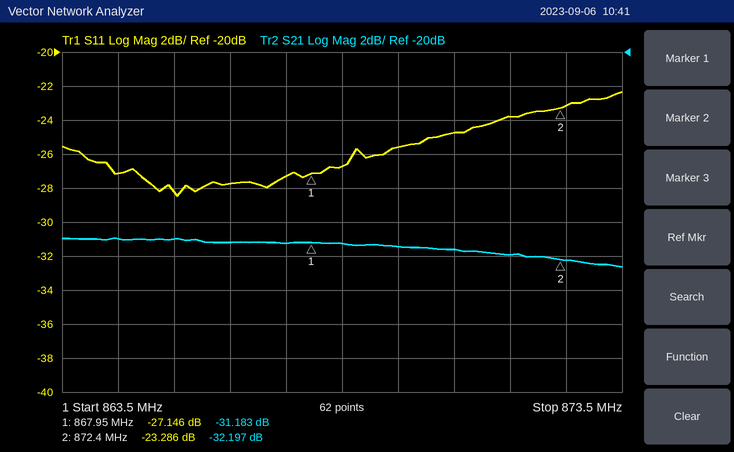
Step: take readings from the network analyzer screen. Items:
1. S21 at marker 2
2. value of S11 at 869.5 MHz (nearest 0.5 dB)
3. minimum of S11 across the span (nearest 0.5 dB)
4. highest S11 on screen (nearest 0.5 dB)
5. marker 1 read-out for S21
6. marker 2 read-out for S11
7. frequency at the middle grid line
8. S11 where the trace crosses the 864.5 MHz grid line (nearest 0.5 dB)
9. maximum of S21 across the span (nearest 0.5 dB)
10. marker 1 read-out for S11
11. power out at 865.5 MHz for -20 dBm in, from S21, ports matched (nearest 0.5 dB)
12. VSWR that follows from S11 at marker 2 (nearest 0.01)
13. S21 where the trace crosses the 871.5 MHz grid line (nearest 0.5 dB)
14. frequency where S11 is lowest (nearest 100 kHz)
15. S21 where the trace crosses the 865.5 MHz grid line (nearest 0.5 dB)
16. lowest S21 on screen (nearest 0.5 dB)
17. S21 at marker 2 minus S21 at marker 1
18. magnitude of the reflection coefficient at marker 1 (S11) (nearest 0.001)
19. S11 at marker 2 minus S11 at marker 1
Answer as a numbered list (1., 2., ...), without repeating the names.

1. -32.197 dB
2. -25.5 dB
3. -28.5 dB
4. -22.5 dB
5. -31.183 dB
6. -23.286 dB
7. 868.5 MHz
8. -27.0 dB
9. -31.0 dB
10. -27.146 dB
11. -51.0 dBm
12. 1.15
13. -32.0 dB
14. 865.6 MHz
15. -31.0 dB
16. -32.5 dB
17. -1.014 dB
18. 0.044
19. 3.860 dB
